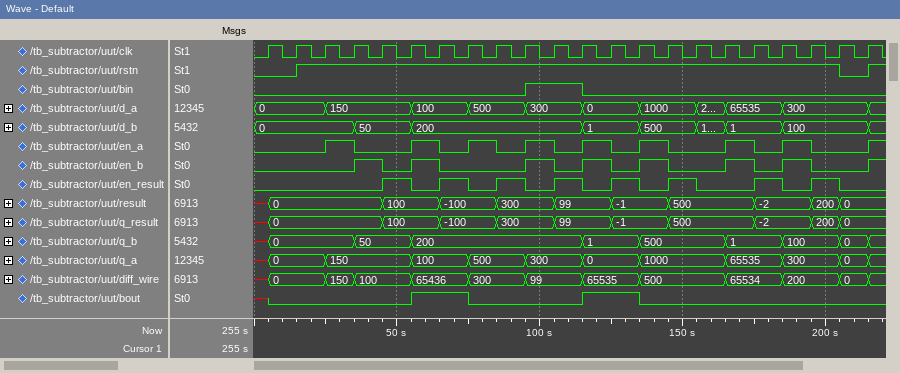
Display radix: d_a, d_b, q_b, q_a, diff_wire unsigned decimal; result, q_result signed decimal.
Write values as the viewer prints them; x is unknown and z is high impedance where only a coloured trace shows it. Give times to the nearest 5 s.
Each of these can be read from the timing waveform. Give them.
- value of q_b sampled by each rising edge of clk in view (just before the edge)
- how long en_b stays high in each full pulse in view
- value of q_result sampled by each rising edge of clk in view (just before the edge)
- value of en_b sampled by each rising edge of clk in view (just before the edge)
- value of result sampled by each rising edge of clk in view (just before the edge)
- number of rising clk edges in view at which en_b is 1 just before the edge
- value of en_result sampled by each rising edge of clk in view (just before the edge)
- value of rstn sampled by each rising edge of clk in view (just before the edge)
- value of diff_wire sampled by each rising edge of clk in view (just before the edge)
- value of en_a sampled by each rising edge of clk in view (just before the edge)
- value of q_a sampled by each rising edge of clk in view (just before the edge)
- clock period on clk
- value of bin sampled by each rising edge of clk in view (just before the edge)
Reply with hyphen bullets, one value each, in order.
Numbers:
- x, 0, 0, 0, 50, 50, 200, 200, 200, 200, 200, 200, 1, 1, 500, 500, 500, 1, 1, 100, 100, 0
- 10 s, 10 s, 10 s, 10 s, 10 s, 10 s, 10 s
- x, 0, 0, 0, 0, 100, 100, -100, -100, 300, 300, 99, 99, -1, -1, 500, 500, 500, -2, -2, 200, 0
- 0 0 0 0 1 0 1 0 0 0 1 0 1 0 1 0 0 1 0 1 0 0
- x, 0, 0, 0, 0, 100, 100, -100, -100, 300, 300, 99, 99, -1, -1, 500, 500, 500, -2, -2, 200, 0
- 7
- 0 0 0 0 0 1 0 1 0 1 0 1 0 1 0 1 0 0 1 0 1 0
- 0 0 1 1 1 1 1 1 1 1 1 1 1 1 1 1 1 1 1 1 1 0
- x, 0, 0, 150, 100, 100, 65436, 65436, 300, 300, 99, 99, 65535, 65535, 500, 500, 500, 65534, 65534, 200, 200, 0
- 0 0 0 1 0 0 1 0 1 0 1 0 1 0 1 0 0 1 0 1 0 0
- x, 0, 0, 150, 150, 150, 100, 100, 500, 500, 300, 300, 0, 0, 1000, 1000, 1000, 65535, 65535, 300, 300, 0
- 10 s
- 0 0 0 0 0 0 0 0 0 0 1 1 0 0 0 0 0 0 0 0 0 0
